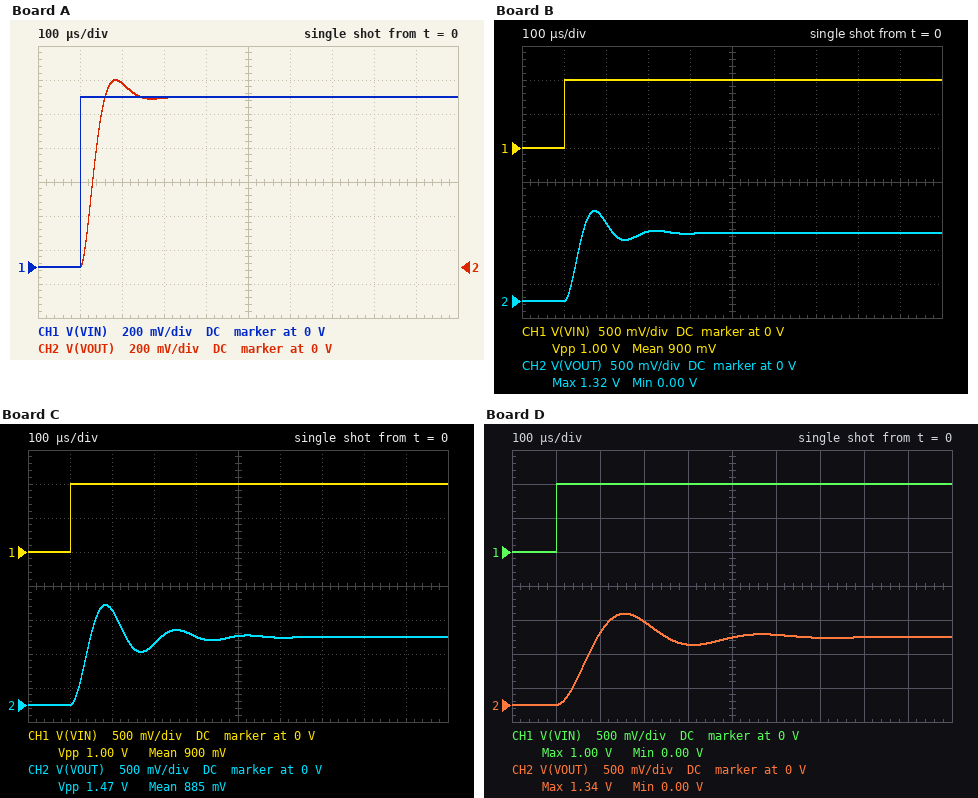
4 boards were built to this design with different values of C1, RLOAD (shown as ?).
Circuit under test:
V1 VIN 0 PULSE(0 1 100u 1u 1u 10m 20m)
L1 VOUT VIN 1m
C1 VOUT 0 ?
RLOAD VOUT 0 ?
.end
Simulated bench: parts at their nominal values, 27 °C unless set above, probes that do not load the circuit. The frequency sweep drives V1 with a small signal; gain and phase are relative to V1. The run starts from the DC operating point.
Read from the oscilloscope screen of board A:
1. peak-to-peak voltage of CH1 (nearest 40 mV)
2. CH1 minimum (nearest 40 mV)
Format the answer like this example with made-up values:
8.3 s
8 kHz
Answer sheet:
1.00 V
0 V
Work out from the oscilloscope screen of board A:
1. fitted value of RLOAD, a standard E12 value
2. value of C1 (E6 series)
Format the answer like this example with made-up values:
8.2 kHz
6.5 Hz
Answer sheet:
39 Ω
470 nF
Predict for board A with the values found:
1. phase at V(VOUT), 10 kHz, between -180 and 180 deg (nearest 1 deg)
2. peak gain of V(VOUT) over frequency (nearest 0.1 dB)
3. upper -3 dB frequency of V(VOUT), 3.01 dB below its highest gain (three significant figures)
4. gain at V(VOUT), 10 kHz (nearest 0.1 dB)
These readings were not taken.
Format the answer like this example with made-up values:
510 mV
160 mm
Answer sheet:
-118 deg
0.4 dB
8.22 kHz
-5.2 dB
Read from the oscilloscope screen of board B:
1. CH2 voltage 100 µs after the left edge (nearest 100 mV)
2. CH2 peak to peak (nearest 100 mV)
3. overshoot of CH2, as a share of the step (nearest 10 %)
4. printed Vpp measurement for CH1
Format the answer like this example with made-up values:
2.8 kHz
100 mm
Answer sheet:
0 V
1.3 V
30 %
1.00 V
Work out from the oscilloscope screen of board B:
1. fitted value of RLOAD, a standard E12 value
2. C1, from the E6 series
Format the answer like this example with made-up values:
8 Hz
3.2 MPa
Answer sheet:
68 Ω
470 nF
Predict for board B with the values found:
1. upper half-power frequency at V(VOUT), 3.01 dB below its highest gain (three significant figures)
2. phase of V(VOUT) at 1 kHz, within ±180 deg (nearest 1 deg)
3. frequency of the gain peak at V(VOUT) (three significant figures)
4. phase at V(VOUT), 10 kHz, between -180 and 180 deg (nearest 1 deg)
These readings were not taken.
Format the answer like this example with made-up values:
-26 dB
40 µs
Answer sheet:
8.71 kHz
-5 deg
6.44 kHz
-133 deg
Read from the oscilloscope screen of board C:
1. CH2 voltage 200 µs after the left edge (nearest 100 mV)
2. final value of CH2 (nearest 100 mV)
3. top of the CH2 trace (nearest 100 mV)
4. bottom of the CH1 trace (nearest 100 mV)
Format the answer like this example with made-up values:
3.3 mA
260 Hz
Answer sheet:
1.4 V
1.0 V
1.5 V
0 V
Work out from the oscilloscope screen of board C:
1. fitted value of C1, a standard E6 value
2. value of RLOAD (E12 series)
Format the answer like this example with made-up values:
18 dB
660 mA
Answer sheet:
680 nF
82 Ω
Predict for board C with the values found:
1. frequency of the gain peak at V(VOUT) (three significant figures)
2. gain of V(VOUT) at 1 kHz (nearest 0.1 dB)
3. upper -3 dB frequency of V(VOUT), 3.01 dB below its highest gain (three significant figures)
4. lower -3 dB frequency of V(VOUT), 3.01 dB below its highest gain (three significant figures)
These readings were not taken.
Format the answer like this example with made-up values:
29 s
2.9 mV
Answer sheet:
5.76 kHz
0.2 dB
7.08 kHz
4.03 kHz
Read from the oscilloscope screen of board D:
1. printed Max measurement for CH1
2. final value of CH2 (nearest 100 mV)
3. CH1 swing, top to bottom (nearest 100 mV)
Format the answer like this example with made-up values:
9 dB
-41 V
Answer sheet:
1.00 V
1.0 V
1.0 V
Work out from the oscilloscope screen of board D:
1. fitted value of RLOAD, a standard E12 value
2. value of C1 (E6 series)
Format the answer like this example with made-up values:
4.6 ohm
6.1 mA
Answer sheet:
33 Ω
2.2 µF
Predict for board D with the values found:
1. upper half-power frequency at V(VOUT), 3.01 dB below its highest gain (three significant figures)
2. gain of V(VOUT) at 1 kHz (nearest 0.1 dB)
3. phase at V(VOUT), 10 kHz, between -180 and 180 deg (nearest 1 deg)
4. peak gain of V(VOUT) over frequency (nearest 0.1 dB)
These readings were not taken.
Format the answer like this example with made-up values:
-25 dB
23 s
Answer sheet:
4.02 kHz
0.6 dB
-166 deg
4.3 dB
